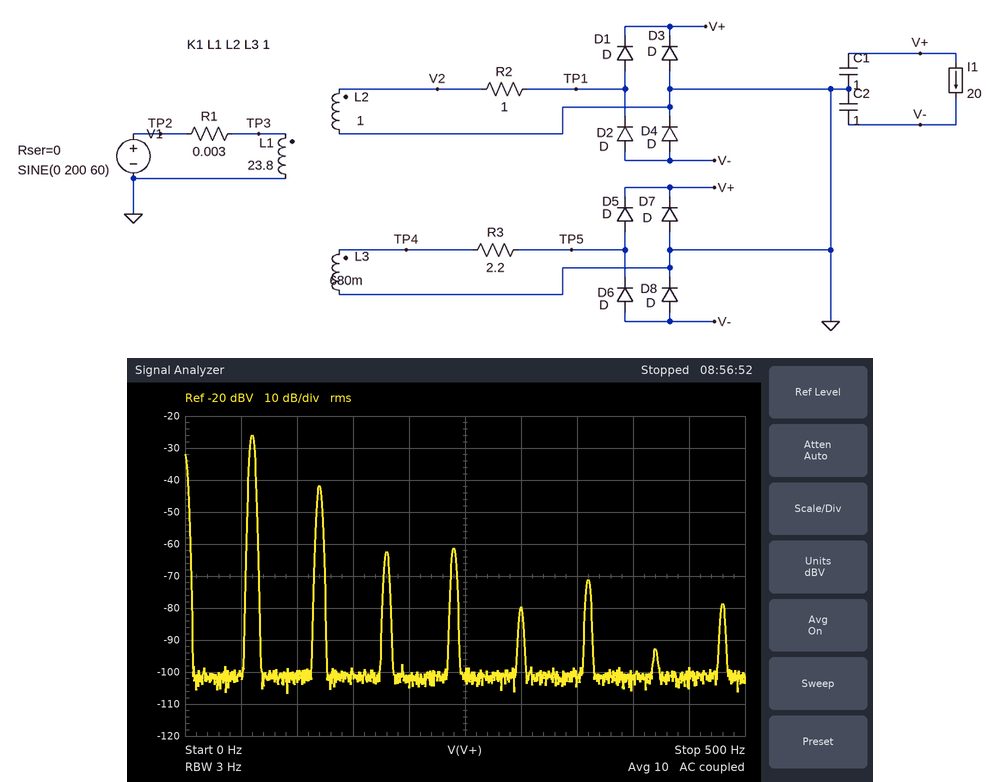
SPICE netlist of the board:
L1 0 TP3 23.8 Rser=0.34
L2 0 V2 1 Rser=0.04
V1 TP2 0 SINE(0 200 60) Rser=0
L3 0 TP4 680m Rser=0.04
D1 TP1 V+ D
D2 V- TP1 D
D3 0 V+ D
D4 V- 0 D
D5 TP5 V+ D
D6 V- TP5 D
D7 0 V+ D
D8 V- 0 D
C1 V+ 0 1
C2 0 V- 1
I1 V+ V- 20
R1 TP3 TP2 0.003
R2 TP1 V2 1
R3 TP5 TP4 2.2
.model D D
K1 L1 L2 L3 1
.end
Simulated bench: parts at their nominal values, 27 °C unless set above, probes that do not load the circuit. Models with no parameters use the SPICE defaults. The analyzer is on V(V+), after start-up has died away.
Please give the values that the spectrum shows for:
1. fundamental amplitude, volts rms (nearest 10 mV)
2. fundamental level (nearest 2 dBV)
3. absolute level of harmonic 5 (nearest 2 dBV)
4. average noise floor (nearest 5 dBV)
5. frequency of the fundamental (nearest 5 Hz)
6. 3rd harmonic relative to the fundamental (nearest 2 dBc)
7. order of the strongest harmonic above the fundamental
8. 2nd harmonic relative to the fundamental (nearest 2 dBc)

50 mV
-26 dBV
-80 dBV
-100 dBV
60 Hz
-36 dBc
2
-16 dBc
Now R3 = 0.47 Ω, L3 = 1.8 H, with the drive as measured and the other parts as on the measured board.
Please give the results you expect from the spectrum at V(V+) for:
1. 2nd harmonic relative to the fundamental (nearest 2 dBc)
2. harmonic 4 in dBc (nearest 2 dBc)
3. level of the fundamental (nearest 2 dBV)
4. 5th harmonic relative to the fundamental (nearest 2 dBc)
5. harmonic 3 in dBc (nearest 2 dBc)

-10 dBc
-56 dBc
-24 dBV
-36 dBc
-22 dBc
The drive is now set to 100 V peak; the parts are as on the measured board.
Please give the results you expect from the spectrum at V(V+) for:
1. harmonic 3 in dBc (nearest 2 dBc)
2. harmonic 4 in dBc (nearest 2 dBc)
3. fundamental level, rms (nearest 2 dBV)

-40 dBc
-40 dBc
-34 dBV
